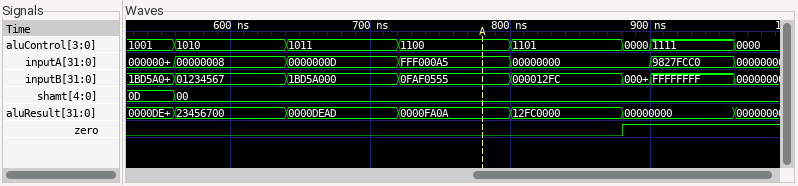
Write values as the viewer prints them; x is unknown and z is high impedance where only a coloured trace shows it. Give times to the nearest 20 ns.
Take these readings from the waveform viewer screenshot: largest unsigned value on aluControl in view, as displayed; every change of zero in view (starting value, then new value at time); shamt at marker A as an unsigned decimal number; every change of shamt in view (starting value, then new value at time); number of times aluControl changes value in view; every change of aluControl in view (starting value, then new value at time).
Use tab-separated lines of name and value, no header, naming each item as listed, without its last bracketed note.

largest unsigned value on aluControl in view, as displayed	1111
every change of zero in view	0, 1 at 880 ns
shamt at marker A as an unsigned decimal number	0
every change of shamt in view	0D, 00 at 560 ns
number of times aluControl changes value in view	7
every change of aluControl in view	1001, 1010 at 560 ns, 1011 at 640 ns, 1100 at 720 ns, 1101 at 800 ns, 0000 at 880 ns, 1111 at 900 ns, 0000 at 960 ns
